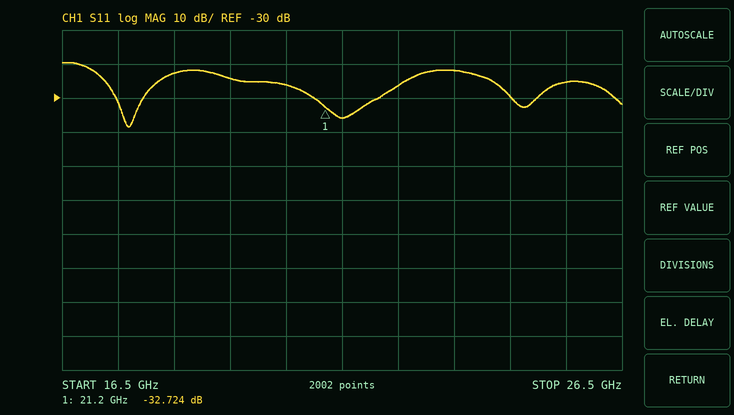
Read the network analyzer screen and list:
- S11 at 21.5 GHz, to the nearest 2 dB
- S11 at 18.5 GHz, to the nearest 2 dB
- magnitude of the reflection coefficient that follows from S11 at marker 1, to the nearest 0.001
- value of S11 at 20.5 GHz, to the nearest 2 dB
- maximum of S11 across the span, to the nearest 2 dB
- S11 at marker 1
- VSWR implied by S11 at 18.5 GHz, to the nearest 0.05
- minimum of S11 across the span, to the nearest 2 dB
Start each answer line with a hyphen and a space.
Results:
- -36 dB
- -22 dB
- 0.023
- -26 dB
- -20 dB
- -32.724 dB
- 1.15
- -38 dB
